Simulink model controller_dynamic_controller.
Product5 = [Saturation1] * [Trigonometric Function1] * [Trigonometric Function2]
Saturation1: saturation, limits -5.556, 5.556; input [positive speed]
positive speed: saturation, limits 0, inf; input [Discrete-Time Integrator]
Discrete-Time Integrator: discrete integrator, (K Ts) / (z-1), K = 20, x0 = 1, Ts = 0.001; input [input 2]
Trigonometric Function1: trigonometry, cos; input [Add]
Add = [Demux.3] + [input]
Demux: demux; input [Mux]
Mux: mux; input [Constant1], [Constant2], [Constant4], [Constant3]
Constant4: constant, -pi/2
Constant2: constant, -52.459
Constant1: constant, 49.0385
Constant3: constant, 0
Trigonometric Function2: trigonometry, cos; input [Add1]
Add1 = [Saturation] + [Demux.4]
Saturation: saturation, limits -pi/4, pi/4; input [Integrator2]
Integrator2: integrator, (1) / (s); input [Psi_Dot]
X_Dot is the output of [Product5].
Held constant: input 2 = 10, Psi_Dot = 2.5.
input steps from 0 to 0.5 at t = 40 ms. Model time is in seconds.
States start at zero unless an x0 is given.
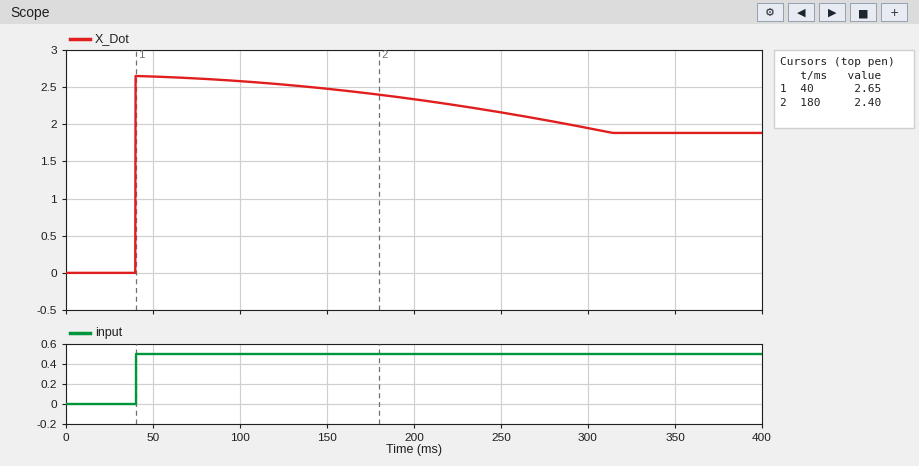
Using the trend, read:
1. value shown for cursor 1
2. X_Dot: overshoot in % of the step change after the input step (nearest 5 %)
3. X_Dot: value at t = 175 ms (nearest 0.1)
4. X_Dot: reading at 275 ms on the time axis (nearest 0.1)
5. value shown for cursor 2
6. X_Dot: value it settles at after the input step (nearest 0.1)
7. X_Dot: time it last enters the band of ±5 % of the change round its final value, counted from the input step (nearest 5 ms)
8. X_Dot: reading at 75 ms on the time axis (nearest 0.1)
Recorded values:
2.65
40 %
2.4
2.1
2.40
1.9
255 ms
2.6
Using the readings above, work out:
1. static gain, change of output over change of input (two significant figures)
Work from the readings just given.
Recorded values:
3.8
